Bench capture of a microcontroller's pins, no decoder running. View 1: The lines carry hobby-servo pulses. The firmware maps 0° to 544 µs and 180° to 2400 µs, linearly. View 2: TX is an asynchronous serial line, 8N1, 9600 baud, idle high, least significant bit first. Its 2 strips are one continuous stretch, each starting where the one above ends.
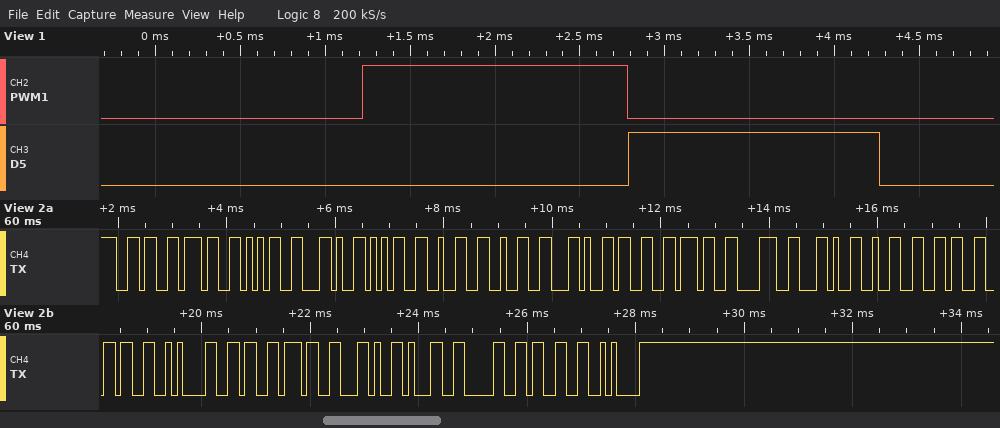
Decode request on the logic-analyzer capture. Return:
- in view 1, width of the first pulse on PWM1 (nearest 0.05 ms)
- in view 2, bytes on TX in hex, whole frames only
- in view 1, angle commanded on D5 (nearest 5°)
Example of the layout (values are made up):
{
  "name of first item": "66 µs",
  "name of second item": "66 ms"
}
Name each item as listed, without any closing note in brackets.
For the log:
{
  "in view 1, width of the first pulse on PWM1": "1.55 ms",
  "in view 2, bytes on TX in hex, whole frames only": "36 37 35 2C 35 32 32 2C 33 37 38 2C 32 36 36 0A 36 37 2C 31 30 33 0A",
  "in view 1, angle commanded on D5": "90°"
}
